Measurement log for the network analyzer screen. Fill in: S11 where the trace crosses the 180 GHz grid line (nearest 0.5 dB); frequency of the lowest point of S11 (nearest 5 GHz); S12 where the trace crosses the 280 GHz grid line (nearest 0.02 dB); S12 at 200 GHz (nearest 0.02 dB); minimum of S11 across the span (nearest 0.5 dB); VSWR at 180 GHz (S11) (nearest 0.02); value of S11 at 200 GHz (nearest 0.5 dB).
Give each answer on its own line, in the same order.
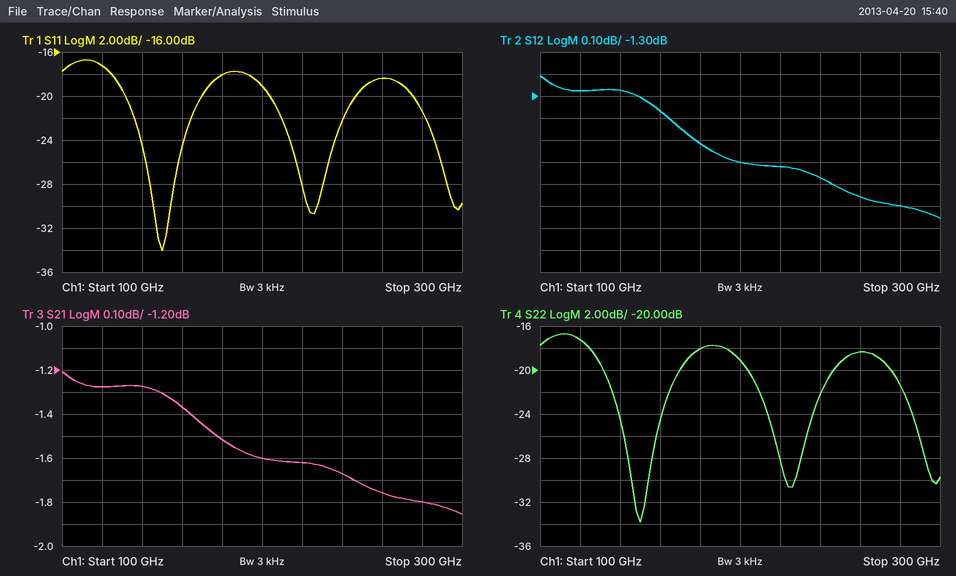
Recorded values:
-18.0 dB
150 GHz
-1.80 dB
-1.60 dB
-34.0 dB
1.28
-19.0 dB
